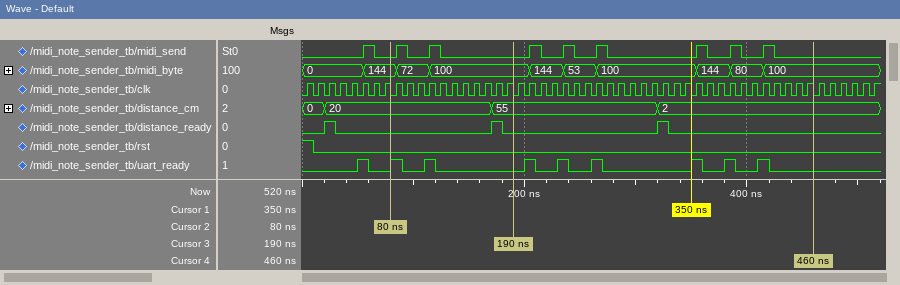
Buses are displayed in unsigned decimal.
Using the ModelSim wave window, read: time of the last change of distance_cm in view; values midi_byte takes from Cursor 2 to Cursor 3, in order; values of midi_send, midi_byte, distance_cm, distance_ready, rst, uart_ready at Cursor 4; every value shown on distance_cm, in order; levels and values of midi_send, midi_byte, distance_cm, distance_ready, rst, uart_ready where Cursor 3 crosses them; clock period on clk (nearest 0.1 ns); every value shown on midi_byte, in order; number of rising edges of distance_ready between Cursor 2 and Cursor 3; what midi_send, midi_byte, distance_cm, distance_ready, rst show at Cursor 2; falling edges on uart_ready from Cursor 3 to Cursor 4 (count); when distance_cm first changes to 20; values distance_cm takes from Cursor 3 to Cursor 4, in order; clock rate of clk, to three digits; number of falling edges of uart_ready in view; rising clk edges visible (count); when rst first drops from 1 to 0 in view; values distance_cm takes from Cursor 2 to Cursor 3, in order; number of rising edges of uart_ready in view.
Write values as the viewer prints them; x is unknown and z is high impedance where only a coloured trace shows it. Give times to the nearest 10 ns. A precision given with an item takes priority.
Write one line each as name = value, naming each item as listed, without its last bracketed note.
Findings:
time of the last change of distance_cm in view = 320 ns
values midi_byte takes from Cursor 2 to Cursor 3, in order = 144, 72, 100
values of midi_send, midi_byte, distance_cm, distance_ready, rst, uart_ready at Cursor 4 = midi_send=0, midi_byte=100, distance_cm=2, distance_ready=0, rst=0, uart_ready=0
every value shown on distance_cm, in order = 0, 20, 55, 2
levels and values of midi_send, midi_byte, distance_cm, distance_ready, rst, uart_ready where Cursor 3 crosses them = midi_send=0, midi_byte=100, distance_cm=55, distance_ready=0, rst=0, uart_ready=0
clock period on clk = 10 ns
every value shown on midi_byte, in order = 0, 144, 72, 100, 144, 53, 100, 144, 80, 100
number of rising edges of distance_ready between Cursor 2 and Cursor 3 = 1
what midi_send, midi_byte, distance_cm, distance_ready, rst show at Cursor 2 = midi_send=0, midi_byte=144, distance_cm=20, distance_ready=0, rst=0
falling edges on uart_ready from Cursor 3 to Cursor 4 = 6
when distance_cm first changes to 20 = 20 ns
values distance_cm takes from Cursor 3 to Cursor 4, in order = 55, 2
clock rate of clk, to three digits = 100 MHz
number of falling edges of uart_ready in view = 9
rising clk edges visible = 52
when rst first drops from 1 to 0 in view = 10 ns
values distance_cm takes from Cursor 2 to Cursor 3, in order = 20, 55
number of rising edges of uart_ready in view = 9
